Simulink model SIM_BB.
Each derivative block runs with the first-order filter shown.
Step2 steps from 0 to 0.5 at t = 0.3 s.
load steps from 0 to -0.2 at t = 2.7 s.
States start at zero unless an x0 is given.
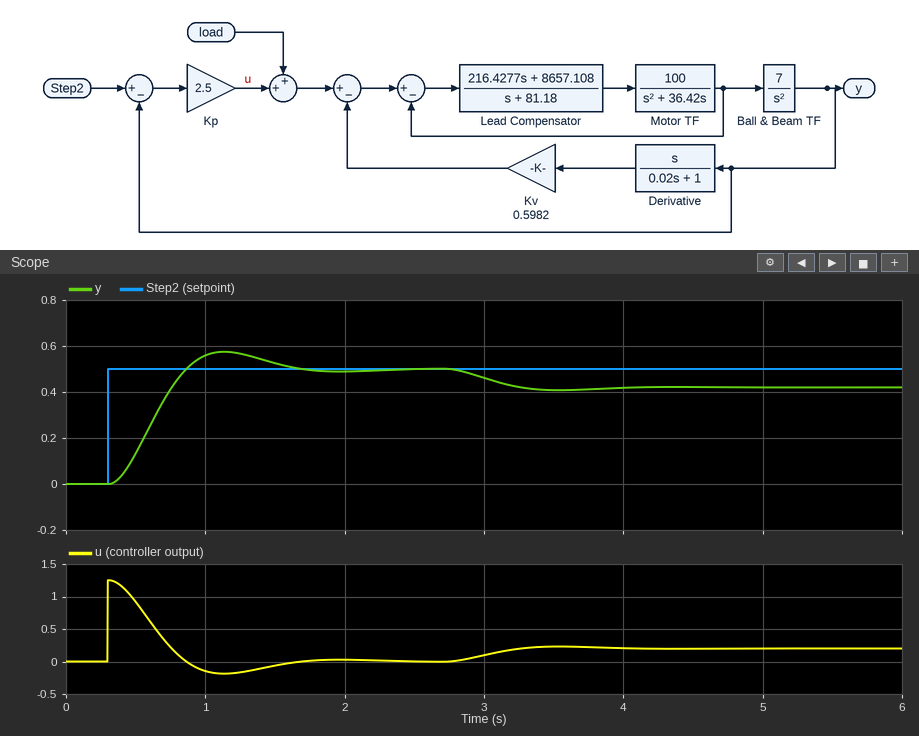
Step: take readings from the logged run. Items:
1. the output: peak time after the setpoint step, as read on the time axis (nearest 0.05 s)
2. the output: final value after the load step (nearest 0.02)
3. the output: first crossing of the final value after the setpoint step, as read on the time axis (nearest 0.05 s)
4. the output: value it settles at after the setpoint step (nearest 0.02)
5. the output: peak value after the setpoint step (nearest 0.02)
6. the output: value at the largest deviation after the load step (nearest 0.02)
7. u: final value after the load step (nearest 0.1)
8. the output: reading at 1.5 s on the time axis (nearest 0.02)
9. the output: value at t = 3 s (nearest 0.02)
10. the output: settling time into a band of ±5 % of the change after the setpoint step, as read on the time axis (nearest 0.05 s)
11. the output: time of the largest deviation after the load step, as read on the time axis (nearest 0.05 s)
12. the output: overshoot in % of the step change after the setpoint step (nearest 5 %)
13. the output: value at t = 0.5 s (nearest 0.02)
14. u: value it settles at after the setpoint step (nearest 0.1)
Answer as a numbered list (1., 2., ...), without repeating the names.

1. 1.15 s
2. 0.42
3. 0.85 s
4. 0.50
5. 0.58
6. 0.40
7. 0.2
8. 0.52
9. 0.46
10. 1.50 s
11. 3.55 s
12. 15 %
13. 0.14
14. 0.0
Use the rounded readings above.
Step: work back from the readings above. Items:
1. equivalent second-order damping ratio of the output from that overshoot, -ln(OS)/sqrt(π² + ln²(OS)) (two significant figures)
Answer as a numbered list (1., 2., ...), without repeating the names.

1. 0.52
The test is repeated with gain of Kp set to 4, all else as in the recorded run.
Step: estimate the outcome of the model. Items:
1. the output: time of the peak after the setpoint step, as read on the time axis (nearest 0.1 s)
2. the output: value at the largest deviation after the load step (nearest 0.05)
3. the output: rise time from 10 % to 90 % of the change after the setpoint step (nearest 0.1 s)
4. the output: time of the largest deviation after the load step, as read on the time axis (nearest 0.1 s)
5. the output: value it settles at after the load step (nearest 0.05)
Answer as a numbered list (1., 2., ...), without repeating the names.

1. 0.9 s
2. 0.45
3. 0.3 s
4. 3.3 s
5. 0.45
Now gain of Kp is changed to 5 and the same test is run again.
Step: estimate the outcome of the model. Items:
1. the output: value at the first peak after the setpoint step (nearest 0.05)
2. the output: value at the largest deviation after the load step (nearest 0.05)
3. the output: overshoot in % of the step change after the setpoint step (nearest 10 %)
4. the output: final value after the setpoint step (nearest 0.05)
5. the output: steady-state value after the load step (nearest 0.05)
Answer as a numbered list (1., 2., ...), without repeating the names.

1. 0.65
2. 0.45
3. 30 %
4. 0.50
5. 0.45
